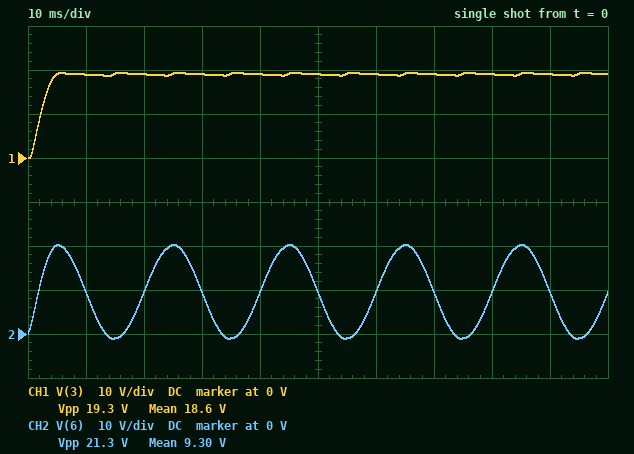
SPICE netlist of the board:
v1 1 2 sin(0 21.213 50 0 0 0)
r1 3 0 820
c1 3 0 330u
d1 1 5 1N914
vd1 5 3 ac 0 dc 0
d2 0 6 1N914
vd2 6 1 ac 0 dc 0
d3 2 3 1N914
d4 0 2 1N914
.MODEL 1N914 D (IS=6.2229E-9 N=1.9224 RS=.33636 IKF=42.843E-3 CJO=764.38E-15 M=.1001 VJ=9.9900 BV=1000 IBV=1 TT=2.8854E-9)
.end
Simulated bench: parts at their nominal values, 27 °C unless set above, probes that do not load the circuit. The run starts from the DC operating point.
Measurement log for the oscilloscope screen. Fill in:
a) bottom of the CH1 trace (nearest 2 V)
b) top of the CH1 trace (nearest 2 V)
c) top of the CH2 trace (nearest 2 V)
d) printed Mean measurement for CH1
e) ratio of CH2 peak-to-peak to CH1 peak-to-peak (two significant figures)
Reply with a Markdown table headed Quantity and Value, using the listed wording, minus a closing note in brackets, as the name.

| Quantity | Value |
|---|---|
| bottom of the CH1 trace | 0 V |
| top of the CH1 trace | 20 V |
| top of the CH2 trace | 20 V |
| printed Mean measurement for CH1 | 18.6 V |
| ratio of CH2 peak-to-peak to CH1 peak-to-peak | 1.1 |
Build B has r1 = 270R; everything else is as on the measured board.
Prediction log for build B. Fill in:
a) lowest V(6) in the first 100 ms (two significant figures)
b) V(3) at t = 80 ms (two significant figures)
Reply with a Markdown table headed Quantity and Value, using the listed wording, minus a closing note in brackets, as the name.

| Quantity | Value |
|---|---|
| lowest V(6) in the first 100 ms | -1.2 V |
| V(3) at t = 80 ms | 18 V |
